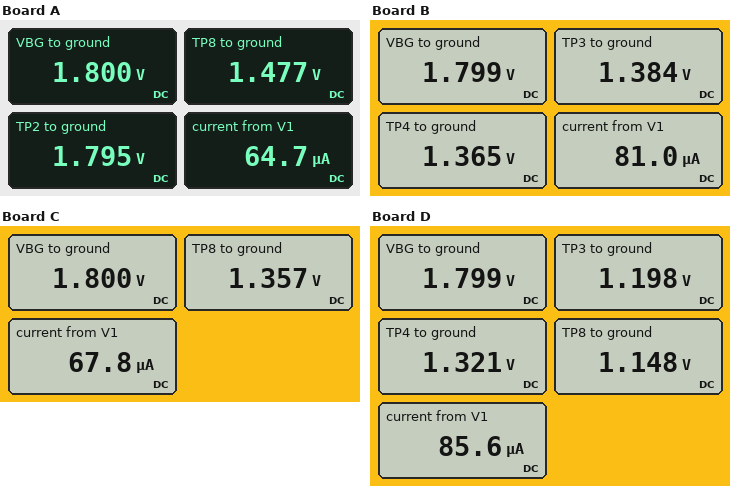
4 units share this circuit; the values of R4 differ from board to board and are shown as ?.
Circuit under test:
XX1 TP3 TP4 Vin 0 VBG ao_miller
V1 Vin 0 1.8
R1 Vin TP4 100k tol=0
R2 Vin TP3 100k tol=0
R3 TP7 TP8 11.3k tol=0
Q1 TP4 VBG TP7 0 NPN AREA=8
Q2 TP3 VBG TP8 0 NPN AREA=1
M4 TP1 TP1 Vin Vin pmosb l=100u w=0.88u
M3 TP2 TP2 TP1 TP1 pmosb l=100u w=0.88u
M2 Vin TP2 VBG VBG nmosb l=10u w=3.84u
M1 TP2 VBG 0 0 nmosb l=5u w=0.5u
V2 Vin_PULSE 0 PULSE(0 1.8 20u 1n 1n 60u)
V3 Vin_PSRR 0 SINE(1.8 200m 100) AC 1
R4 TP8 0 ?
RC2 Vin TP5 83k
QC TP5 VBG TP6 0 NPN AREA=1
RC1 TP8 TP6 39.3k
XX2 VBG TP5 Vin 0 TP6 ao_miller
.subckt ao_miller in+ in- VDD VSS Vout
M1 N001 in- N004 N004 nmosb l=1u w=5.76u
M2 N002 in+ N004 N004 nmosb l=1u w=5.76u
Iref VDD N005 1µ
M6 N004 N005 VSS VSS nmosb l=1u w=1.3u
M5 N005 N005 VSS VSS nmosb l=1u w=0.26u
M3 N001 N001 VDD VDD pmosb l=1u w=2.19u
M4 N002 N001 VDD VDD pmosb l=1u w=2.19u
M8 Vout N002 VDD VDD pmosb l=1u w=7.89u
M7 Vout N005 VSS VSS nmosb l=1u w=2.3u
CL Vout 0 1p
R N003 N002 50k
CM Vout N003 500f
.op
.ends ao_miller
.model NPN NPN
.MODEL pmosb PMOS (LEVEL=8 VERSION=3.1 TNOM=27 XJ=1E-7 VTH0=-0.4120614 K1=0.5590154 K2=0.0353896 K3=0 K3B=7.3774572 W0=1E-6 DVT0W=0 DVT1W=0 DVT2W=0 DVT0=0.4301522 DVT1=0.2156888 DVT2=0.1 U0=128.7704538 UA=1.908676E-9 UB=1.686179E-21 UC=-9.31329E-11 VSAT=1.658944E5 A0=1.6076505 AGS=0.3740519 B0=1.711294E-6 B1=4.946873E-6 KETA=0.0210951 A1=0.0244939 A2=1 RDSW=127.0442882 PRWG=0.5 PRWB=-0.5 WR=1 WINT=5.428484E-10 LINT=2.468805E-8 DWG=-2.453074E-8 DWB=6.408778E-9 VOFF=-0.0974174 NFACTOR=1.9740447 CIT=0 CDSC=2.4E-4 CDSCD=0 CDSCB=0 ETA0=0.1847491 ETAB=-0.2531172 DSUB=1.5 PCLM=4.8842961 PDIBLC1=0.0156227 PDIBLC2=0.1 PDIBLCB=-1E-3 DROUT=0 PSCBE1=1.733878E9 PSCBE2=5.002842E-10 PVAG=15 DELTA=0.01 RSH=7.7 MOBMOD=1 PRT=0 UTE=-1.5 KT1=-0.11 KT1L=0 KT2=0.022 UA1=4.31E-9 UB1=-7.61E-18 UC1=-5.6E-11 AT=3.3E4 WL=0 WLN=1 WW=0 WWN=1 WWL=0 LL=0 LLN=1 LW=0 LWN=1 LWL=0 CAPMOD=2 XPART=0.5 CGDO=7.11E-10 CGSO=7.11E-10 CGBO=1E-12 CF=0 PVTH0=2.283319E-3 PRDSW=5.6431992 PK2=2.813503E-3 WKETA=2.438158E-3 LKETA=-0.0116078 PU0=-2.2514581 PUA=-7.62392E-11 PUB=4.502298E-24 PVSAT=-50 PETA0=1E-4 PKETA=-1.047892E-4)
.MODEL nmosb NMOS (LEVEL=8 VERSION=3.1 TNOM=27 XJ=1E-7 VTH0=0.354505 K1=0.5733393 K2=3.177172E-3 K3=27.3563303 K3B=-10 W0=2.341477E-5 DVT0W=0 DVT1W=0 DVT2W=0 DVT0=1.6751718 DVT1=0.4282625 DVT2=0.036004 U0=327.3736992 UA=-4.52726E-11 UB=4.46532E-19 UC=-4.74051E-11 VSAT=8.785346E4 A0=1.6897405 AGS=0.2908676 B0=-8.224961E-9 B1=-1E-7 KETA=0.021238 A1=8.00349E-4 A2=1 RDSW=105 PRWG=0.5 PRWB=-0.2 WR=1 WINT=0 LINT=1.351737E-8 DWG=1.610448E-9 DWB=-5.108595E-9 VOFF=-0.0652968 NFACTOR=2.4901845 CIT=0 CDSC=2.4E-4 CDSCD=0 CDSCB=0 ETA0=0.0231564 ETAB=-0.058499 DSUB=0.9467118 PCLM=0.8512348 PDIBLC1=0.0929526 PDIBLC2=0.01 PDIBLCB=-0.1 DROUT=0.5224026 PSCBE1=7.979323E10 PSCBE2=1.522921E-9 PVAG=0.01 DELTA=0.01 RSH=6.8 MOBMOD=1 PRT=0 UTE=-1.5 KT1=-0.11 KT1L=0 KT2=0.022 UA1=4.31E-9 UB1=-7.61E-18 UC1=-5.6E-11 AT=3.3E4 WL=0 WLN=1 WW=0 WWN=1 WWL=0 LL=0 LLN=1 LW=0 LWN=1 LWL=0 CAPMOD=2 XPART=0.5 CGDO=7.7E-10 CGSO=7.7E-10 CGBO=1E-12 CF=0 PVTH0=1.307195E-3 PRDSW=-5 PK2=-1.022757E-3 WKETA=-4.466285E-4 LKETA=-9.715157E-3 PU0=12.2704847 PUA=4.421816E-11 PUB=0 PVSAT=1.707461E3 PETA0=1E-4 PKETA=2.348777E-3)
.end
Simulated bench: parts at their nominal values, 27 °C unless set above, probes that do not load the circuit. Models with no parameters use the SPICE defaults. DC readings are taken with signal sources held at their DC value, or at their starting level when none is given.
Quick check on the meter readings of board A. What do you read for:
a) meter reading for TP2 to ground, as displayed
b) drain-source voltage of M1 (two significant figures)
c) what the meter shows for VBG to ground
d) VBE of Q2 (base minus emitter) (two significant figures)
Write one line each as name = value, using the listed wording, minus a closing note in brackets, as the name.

meter reading for TP2 to ground, as displayed = 1.795 V
drain-source voltage of M1 = 1.8 V
what the meter shows for VBG to ground = 1.800 V
VBE of Q2 (base minus emitter) = 320 mV
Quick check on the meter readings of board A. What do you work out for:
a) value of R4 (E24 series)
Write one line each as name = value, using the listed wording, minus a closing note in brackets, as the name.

value of R4 = 180 kΩ
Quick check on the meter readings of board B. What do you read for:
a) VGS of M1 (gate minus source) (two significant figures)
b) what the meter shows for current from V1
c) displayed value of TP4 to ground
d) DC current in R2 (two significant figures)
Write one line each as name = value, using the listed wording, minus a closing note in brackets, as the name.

VGS of M1 (gate minus source) = 1.8 V
what the meter shows for current from V1 = 81.0 µA
displayed value of TP4 to ground = 1.365 V
DC current in R2 = 4.2 µA
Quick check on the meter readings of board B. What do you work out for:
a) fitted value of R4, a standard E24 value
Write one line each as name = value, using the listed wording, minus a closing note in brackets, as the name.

fitted value of R4, a standard E24 value = 47 kΩ
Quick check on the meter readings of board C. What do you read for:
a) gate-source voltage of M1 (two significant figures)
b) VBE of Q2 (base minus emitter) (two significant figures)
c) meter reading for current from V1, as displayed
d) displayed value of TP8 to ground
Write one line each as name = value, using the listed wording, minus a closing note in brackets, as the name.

gate-source voltage of M1 = 1.8 V
VBE of Q2 (base minus emitter) = 440 mV
meter reading for current from V1, as displayed = 67.8 µA
displayed value of TP8 to ground = 1.357 V
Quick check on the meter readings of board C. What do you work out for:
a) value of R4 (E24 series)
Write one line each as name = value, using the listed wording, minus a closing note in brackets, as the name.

value of R4 = 120 kΩ
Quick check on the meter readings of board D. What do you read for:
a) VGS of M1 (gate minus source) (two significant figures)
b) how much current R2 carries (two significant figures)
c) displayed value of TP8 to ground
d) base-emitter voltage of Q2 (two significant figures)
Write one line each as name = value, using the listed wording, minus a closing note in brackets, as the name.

VGS of M1 (gate minus source) = 1.8 V
how much current R2 carries = 6.0 µA
displayed value of TP8 to ground = 1.148 V
base-emitter voltage of Q2 = 650 mV
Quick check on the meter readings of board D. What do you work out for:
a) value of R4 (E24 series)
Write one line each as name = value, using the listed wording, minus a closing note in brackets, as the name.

value of R4 = 39 kΩ
